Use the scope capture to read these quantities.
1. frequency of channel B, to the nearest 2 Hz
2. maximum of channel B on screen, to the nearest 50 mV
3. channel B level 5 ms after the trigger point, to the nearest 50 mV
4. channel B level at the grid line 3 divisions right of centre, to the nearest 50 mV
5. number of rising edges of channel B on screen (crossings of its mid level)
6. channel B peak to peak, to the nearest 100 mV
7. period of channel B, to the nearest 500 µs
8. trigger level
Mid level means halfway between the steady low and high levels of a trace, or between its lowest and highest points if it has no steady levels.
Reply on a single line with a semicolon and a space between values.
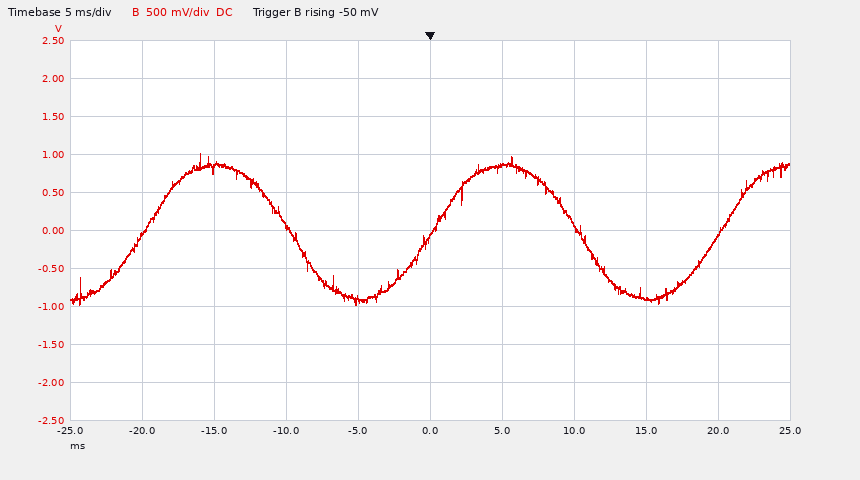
50 Hz; 1.00 V; 850 mV; -900 mV; 3; 2.00 V; 20.0 ms; -50 mV
